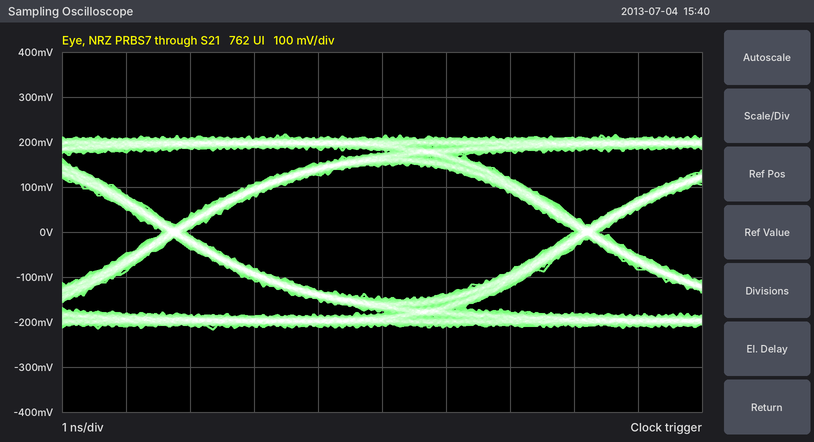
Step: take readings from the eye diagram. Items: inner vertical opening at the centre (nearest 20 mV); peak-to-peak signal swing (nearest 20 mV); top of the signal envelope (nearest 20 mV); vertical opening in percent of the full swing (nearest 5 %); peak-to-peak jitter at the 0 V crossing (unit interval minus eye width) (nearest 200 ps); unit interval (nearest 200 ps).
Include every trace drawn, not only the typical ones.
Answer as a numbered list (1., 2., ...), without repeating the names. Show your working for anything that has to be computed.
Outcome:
1. 300 mV
2. 440 mV
3. 220 mV
4. 300 mV / 440 mV ≈ 68.2 %, so 70 % to the nearest 5 %
5. 400 ps
6. 6.4 ns
